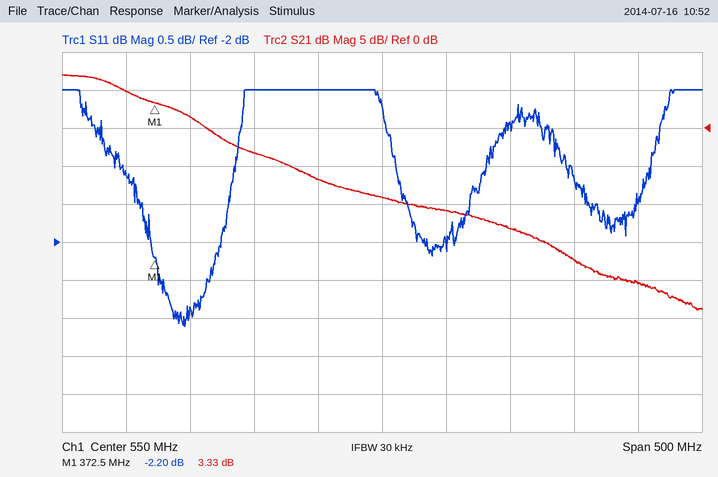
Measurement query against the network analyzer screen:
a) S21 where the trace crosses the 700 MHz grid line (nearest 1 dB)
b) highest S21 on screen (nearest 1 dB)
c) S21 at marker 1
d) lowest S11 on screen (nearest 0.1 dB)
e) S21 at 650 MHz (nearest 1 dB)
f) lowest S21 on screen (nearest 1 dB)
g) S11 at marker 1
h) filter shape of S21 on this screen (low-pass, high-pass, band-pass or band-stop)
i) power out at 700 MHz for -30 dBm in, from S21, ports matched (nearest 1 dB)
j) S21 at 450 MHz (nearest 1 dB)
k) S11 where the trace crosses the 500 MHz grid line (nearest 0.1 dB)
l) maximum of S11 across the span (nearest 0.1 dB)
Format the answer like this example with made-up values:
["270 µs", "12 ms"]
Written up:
["-17 dB", "7 dB", "3.33 dB", "-3.1 dB", "-13 dB", "-24 dB", "-2.20 dB", "low-pass", "-47 dBm", "-3 dB", "0.0 dB", "0.0 dB"]
